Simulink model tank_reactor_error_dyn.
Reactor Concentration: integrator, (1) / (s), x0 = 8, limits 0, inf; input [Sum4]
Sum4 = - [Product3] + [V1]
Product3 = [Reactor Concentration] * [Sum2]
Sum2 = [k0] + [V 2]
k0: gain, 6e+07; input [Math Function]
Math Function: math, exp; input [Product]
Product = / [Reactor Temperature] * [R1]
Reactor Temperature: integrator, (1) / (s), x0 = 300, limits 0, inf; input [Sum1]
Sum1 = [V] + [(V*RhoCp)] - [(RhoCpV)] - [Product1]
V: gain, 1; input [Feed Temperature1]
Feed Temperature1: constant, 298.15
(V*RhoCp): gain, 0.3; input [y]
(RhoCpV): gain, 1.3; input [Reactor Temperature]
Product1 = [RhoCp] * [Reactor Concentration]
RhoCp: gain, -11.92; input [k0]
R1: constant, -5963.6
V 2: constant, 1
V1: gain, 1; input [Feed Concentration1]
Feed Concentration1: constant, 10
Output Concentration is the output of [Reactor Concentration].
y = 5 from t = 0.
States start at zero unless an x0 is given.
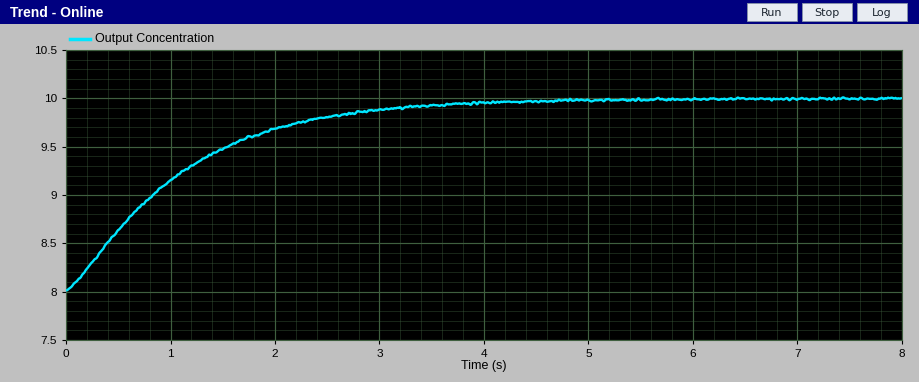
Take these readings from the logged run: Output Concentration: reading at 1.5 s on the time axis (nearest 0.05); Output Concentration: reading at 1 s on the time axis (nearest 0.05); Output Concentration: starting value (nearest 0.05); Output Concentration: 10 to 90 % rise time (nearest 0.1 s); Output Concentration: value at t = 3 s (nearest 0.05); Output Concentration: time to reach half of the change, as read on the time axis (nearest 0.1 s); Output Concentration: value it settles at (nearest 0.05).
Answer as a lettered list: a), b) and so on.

a) 9.50
b) 9.15
c) 8.00
d) 2.3 s
e) 9.90
f) 0.8 s
g) 10.00
